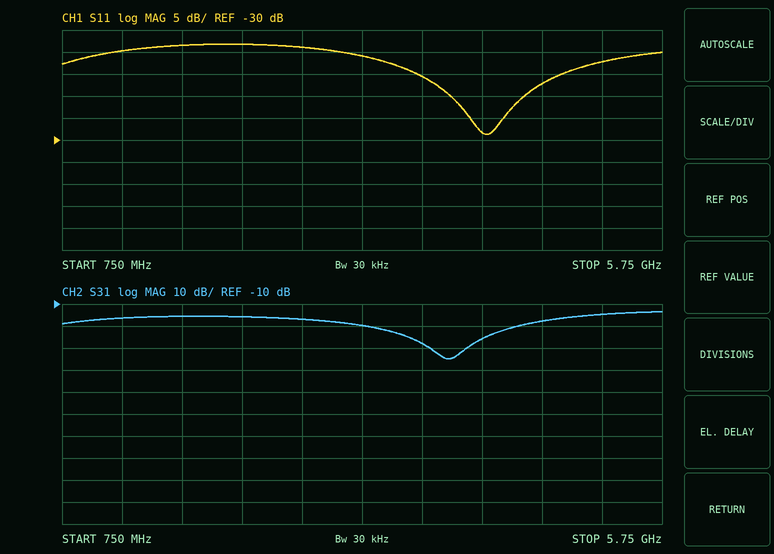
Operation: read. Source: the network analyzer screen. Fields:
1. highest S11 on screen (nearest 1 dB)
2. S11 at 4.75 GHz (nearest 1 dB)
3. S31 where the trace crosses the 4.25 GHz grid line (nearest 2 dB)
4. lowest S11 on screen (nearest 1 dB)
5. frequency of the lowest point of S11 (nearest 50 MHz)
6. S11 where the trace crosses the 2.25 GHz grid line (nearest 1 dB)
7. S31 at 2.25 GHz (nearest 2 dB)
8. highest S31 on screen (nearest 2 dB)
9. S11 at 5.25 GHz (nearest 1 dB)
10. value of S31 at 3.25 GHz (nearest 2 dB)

-8 dB
-17 dB
-26 dB
-29 dB
4.30 GHz
-8 dB
-16 dB
-14 dB
-12 dB
-20 dB
